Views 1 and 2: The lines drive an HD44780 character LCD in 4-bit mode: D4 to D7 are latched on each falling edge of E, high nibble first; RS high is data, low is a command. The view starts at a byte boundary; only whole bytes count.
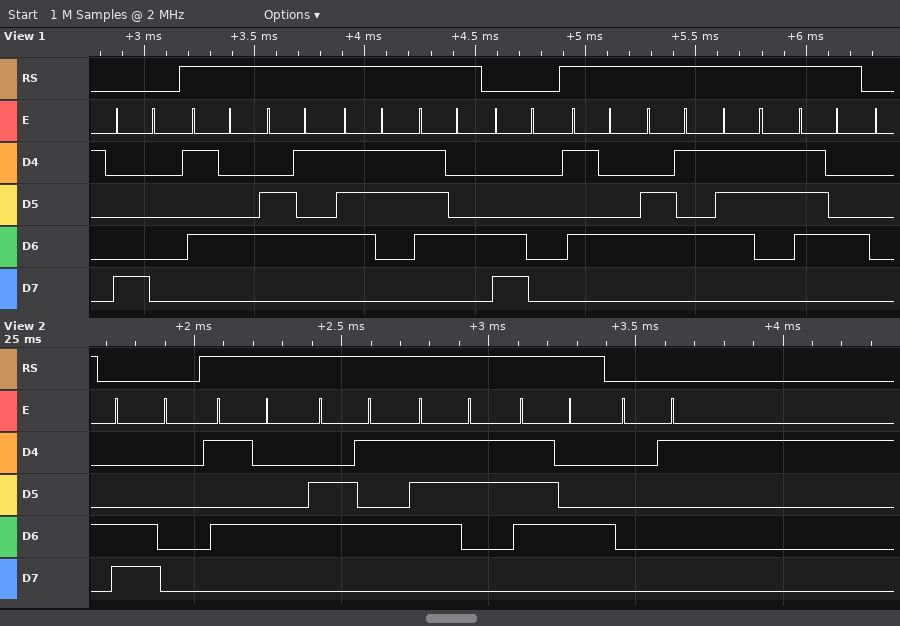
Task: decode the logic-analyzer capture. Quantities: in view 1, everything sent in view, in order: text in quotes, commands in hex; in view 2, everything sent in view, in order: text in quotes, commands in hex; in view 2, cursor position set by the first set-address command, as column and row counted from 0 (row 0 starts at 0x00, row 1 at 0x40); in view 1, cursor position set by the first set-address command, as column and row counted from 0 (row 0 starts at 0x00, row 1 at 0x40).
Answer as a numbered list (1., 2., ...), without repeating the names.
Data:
1. 0x80 "Test" 0xC0 "Test"
2. 0xC0 "Test" 0x01
3. column 0, row 1
4. column 0, row 0
